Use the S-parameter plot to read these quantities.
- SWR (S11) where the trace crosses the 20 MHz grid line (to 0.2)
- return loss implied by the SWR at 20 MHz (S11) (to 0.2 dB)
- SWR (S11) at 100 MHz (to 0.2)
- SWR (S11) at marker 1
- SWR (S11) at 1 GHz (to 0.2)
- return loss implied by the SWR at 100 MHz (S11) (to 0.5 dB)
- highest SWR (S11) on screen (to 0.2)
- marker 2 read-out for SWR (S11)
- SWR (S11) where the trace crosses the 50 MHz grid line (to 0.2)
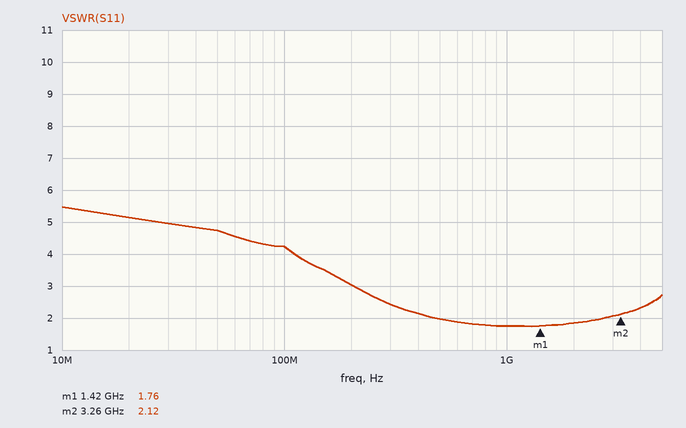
5.2
3.4 dB
4.2
1.76
1.8
4.0 dB
5.4
2.12
4.8
